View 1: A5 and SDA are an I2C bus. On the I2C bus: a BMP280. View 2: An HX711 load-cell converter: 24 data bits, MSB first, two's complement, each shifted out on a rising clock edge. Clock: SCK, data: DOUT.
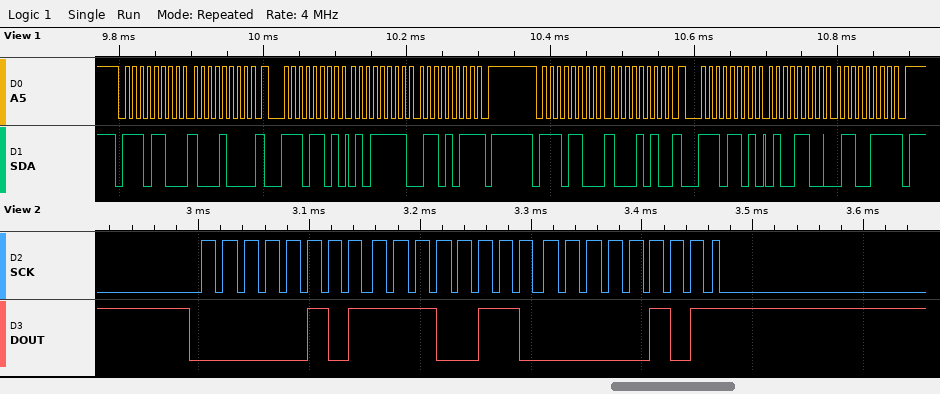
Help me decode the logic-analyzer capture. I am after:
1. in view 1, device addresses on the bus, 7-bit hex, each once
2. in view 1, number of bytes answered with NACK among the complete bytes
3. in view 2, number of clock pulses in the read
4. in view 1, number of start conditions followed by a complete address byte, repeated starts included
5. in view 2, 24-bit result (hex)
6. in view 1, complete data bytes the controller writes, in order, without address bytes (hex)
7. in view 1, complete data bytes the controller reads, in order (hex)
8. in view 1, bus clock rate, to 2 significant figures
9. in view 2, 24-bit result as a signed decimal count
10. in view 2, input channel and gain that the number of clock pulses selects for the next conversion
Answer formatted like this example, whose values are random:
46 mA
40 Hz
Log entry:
0x76
2
25
4
0x05E605
88 8A
5F 6B 4C 67
100 kHz
386565
channel A, gain 128
